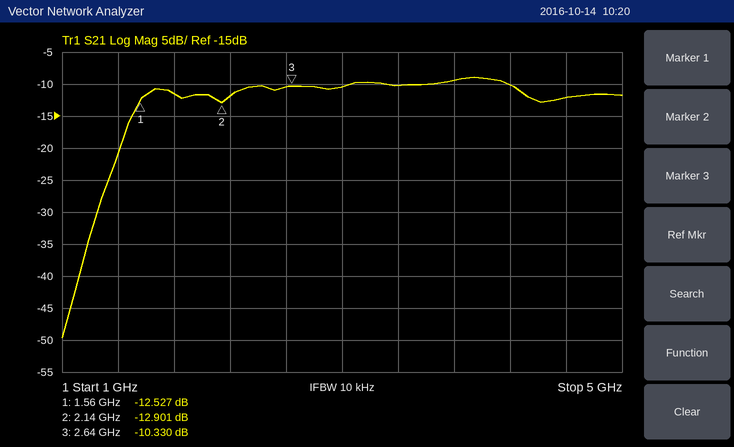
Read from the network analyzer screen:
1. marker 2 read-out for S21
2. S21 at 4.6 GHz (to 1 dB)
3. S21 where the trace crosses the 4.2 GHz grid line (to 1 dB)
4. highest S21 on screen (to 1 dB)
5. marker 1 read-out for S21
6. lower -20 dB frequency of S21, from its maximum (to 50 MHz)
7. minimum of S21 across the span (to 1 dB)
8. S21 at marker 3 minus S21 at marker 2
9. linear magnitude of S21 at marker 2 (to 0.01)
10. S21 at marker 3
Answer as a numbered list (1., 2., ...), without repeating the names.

1. -12.901 dB
2. -12 dB
3. -10 dB
4. -9 dB
5. -12.527 dB
6. 1.25 GHz
7. -50 dB
8. 2.571 dB
9. 0.23
10. -10.330 dB
